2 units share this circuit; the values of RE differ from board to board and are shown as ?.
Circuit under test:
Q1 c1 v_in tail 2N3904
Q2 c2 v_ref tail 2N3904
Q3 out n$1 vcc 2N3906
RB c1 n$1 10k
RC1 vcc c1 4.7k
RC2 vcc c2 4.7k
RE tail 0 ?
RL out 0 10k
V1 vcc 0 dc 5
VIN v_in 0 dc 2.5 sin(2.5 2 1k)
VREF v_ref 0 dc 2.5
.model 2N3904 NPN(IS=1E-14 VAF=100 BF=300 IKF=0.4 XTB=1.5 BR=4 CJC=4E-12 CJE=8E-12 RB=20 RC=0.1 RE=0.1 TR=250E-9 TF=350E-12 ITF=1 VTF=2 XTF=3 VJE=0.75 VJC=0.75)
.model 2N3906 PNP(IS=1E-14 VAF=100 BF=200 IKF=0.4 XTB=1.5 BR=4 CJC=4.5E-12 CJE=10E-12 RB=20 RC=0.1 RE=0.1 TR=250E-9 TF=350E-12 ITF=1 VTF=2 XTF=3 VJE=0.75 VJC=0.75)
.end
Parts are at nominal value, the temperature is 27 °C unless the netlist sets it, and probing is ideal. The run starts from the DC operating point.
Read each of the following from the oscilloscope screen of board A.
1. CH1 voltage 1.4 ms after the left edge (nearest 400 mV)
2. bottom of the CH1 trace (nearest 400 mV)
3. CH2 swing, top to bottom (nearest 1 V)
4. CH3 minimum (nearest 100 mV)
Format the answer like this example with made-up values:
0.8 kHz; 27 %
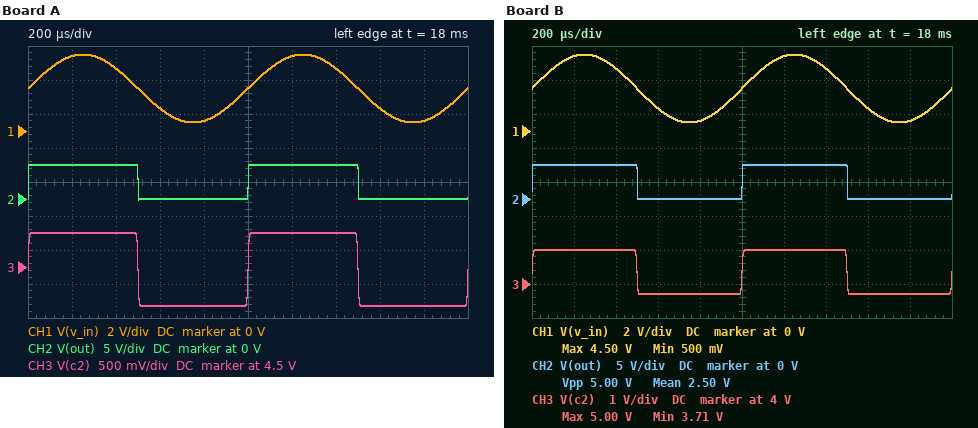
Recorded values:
3.6 V; 400 mV; 5 V; 3.9 V
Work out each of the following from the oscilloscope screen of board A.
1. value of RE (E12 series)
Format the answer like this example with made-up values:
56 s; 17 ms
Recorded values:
8.2 kΩ
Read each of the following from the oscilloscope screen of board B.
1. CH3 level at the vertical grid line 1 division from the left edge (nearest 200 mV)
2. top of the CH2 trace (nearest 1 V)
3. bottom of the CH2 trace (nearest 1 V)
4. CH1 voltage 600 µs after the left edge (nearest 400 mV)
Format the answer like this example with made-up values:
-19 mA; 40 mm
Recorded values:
5.0 V; 5 V; 0 V; 1.2 V
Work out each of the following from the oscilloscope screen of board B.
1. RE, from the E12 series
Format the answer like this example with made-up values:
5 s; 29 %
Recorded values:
6.8 kΩ
